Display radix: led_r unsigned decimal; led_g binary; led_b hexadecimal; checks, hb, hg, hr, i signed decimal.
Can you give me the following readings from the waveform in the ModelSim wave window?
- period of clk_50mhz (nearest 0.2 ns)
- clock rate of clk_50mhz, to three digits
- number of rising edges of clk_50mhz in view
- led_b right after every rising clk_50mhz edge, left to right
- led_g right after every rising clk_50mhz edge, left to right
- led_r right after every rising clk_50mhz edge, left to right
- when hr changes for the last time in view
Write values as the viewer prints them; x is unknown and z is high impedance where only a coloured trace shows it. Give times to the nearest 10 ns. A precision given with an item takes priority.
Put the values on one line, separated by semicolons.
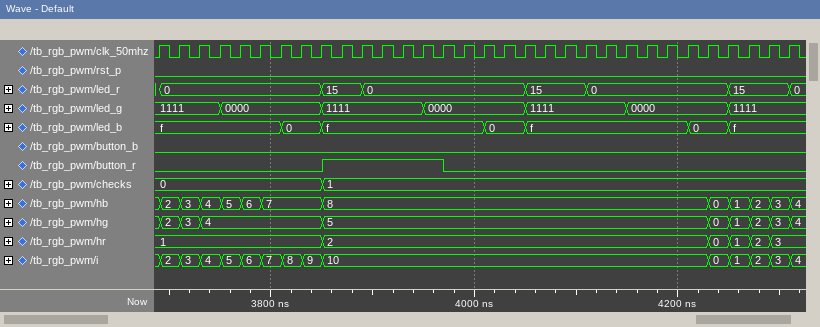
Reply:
20 ns; 50.0 MHz; 32; f, f, f, f, f, f, 0, 0, f, f, f, f, f, f, f, f, 0, 0, f, f, f, f, f, f, f, f, 0, 0, f, f, f, f; 1111, 1111, 1111, 0000, 0000, 0000, 0000, 0000, 1111, 1111, 1111, 1111, 1111, 0000, 0000, 0000, 0000, 0000, 1111, 1111, 1111, 1111, 1111, 0000, 0000, 0000, 0000, 0000, 1111, 1111, 1111, 1111; 0, 0, 0, 0, 0, 0, 0, 0, 15, 15, 0, 0, 0, 0, 0, 0, 0, 0, 15, 15, 15, 0, 0, 0, 0, 0, 0, 0, 15, 15, 15, 0; 4290 ns
